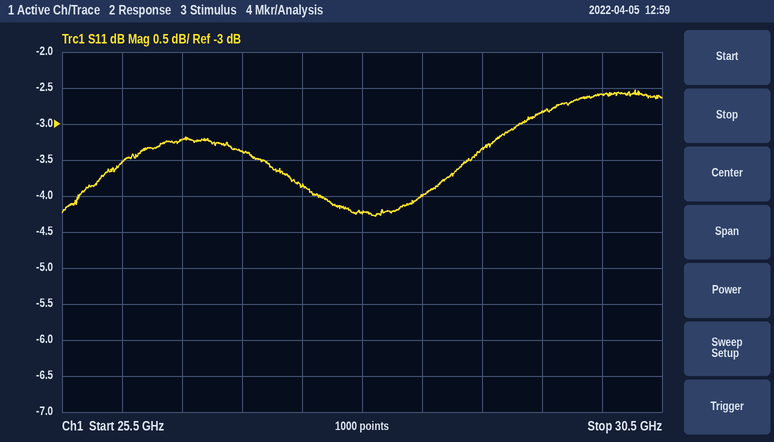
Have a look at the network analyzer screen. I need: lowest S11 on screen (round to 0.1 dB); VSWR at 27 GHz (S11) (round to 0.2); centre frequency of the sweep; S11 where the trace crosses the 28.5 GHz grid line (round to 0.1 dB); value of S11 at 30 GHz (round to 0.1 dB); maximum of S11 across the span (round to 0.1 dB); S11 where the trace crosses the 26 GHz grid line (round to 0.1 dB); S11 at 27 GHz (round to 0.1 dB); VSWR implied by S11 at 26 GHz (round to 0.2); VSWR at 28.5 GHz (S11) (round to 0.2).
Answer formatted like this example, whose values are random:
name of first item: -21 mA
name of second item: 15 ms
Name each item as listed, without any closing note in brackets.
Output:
lowest S11 on screen: -4.3 dB
VSWR at 27 GHz (S11): 5.2
centre frequency of the sweep: 28 GHz
S11 where the trace crosses the 28.5 GHz grid line: -4.0 dB
value of S11 at 30 GHz: -2.6 dB
maximum of S11 across the span: -2.5 dB
S11 where the trace crosses the 26 GHz grid line: -3.5 dB
S11 at 27 GHz: -3.4 dB
VSWR implied by S11 at 26 GHz: 5.0
VSWR at 28.5 GHz (S11): 4.4
